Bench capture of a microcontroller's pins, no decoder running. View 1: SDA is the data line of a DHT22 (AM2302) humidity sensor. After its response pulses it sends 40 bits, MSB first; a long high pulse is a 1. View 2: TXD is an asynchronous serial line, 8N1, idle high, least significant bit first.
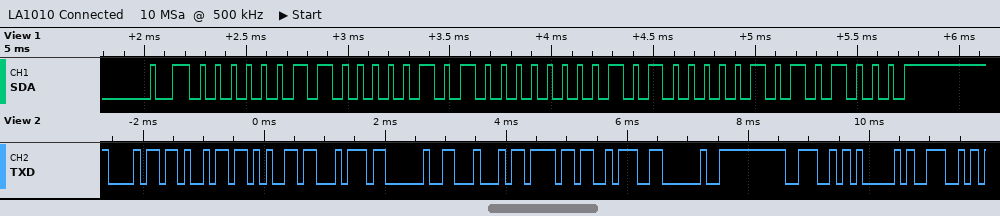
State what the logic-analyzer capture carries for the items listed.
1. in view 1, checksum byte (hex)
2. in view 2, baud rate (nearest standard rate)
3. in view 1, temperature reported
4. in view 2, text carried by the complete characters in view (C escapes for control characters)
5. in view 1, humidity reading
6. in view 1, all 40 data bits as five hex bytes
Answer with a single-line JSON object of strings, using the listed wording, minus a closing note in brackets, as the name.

{"in view 1, checksum byte": "0xA8", "in view 2, baud rate": "9600 baud", "in view 1, temperature reported": "16.0 °C", "in view 2, text carried by the complete characters in view": "\"hiet Do: NAN\"", "in view 1, humidity reading": "77.3 %", "in view 1, all 40 data bits as five hex bytes": "03 05 00 A0 A8"}
